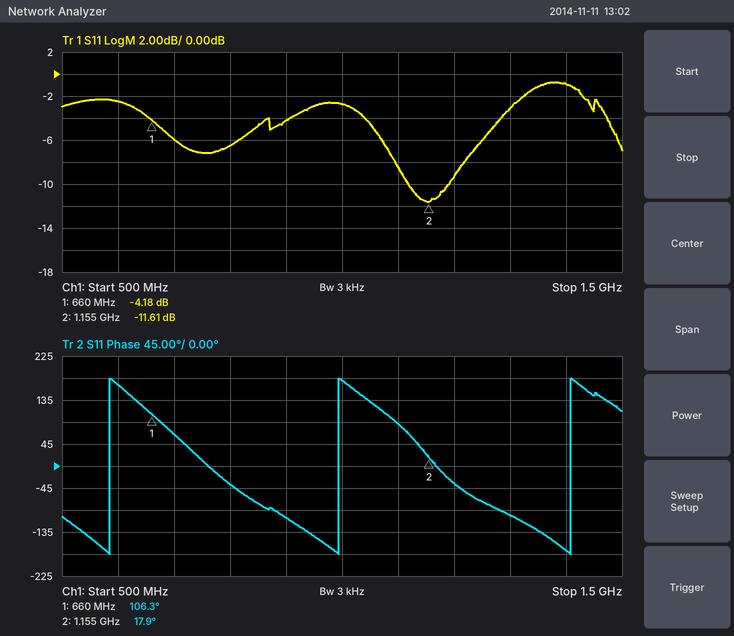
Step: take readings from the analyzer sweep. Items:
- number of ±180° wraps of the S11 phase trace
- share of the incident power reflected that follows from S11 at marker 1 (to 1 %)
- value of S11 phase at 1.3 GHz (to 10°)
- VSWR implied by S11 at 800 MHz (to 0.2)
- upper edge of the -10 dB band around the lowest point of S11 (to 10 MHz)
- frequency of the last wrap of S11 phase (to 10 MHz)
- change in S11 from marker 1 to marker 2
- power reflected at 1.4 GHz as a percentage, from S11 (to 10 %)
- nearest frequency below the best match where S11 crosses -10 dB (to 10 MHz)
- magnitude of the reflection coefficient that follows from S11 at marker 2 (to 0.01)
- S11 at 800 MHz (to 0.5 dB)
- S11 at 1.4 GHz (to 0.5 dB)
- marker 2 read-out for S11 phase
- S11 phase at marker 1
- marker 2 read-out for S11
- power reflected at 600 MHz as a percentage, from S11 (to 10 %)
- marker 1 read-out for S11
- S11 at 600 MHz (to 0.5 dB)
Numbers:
3
38 %
-100°
2.8
1.19 GHz
1.41 GHz
-7.43 dB
80 %
1.12 GHz
0.26
-6.5 dB
-1.0 dB
17.9°
106.3°
-11.61 dB
60 %
-4.18 dB
-2.5 dB
